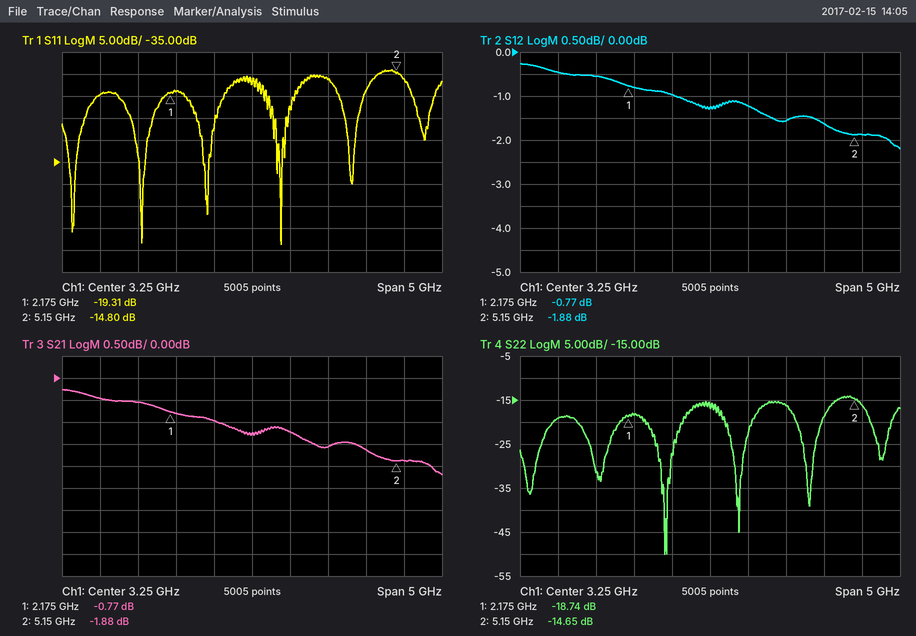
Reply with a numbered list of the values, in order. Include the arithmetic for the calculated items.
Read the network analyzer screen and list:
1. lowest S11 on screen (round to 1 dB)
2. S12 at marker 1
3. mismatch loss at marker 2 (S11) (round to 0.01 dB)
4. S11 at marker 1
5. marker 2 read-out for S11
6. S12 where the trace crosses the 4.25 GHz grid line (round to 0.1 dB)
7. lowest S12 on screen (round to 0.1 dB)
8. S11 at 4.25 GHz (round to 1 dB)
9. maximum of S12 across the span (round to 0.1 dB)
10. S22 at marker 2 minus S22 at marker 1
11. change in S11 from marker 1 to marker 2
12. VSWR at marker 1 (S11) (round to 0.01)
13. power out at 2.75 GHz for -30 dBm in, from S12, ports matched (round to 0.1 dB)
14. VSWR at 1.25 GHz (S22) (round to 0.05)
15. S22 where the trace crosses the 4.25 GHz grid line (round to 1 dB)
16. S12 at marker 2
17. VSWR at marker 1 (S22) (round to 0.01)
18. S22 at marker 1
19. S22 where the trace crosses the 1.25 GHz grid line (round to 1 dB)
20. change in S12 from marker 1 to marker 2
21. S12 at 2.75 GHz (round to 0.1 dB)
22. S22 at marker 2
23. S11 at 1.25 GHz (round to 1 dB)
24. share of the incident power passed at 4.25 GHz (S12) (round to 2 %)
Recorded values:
1. -54 dB
2. -0.77 dB
3. −10 log10(1 − 10^(-14.8/10)) ≈ 0.15 dB
4. -19.31 dB
5. -14.80 dB
6. -1.6 dB
7. -2.2 dB
8. -16 dB
9. -0.3 dB
10. -14.65 − (-18.74) = 4.09 dB
11. -14.8 − (-19.31) = 4.51 dB
12. (1 + 0.1083)/(1 − 0.1083) ≈ 1.24
13. -30 dBm + (-1.0 dB) = -31.0 dBm
14. |Γ| = 10^(-19/20) = 0.1122; VSWR = (1 + 0.1122)/(1 − 0.1122) ≈ 1.25
15. -16 dB
16. -1.88 dB
17. (1 + 0.1156)/(1 − 0.1156) ≈ 1.26
18. -18.74 dB
19. -19 dB
20. -1.88 − (-0.77) = -1.11 dB
21. -1.0 dB
22. -14.65 dB
23. -20 dB
24. 10^(-1.6/10) ≈ 69.2 %, so 70 % to the nearest 2 %
